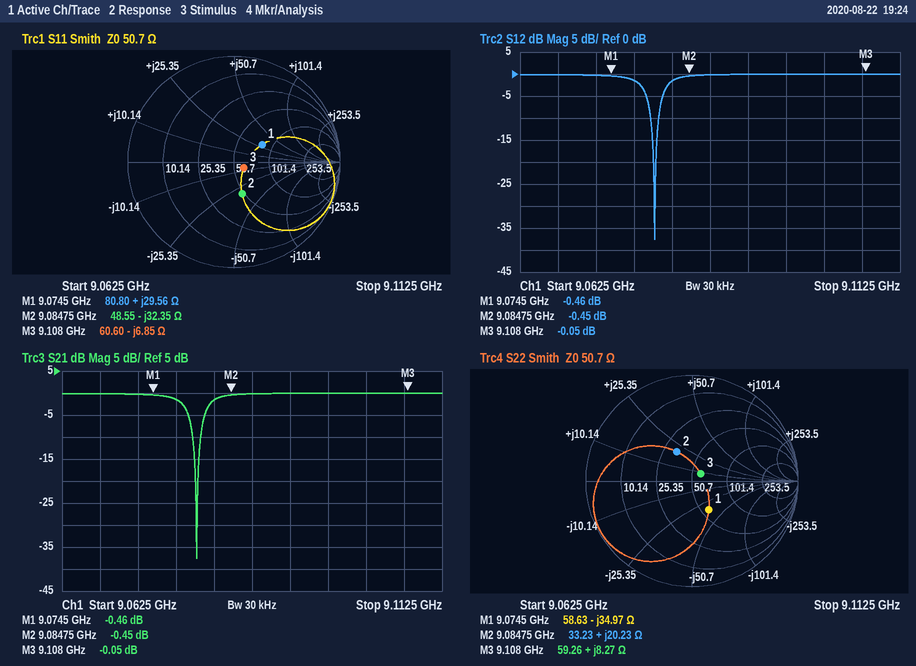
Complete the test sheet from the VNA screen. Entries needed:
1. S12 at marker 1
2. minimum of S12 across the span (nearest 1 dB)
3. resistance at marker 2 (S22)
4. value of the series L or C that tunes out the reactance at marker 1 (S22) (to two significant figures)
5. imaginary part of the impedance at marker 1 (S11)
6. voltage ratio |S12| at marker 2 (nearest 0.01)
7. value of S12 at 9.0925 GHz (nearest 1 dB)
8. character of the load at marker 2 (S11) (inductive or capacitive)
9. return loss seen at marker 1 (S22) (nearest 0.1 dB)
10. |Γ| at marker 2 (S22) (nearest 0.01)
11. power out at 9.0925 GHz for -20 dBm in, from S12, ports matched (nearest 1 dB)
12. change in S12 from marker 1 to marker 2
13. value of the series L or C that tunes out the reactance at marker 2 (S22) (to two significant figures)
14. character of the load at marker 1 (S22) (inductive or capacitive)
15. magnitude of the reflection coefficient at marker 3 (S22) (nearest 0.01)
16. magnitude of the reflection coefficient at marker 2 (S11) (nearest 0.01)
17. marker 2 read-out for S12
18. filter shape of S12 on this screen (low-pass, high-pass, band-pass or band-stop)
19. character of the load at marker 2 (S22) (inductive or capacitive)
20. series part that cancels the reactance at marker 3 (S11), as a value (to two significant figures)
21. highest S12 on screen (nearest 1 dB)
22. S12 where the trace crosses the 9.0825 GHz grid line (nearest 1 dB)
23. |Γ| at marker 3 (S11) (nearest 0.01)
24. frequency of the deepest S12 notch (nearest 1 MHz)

-0.46 dB
-38 dB
33.23 Ω
610 pH
+29.56 Ω
0.95
0 dB
capacitive
10.1 dB
0.31
-20 dBm
0.01 dB
870 fF
capacitive
0.11
0.31
-0.45 dB
band-stop
inductive
120 pH
0 dB
-2 dB
0.11
9.080 GHz
